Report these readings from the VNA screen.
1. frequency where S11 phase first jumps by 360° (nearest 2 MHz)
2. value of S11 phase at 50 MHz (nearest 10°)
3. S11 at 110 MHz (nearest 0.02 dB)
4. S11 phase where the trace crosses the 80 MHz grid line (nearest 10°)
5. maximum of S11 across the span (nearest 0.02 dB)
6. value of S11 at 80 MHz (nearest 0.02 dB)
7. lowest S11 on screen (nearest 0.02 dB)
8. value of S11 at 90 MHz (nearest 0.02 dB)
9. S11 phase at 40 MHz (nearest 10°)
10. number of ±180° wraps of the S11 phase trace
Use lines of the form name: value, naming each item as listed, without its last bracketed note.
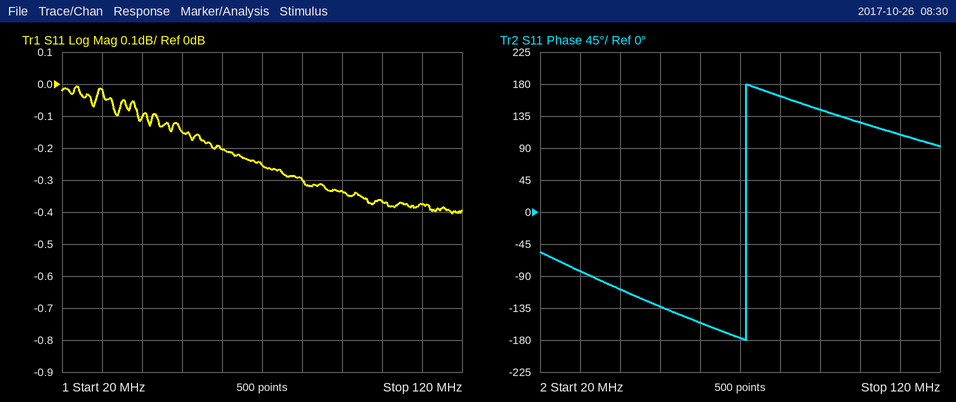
frequency where S11 phase first jumps by 360°: 72 MHz
value of S11 phase at 50 MHz: -130°
S11 at 110 MHz: -0.38 dB
S11 phase where the trace crosses the 80 MHz grid line: 160°
maximum of S11 across the span: 0.00 dB
value of S11 at 80 MHz: -0.30 dB
lowest S11 on screen: -0.40 dB
value of S11 at 90 MHz: -0.34 dB
S11 phase at 40 MHz: -110°
number of ±180° wraps of the S11 phase trace: 1
